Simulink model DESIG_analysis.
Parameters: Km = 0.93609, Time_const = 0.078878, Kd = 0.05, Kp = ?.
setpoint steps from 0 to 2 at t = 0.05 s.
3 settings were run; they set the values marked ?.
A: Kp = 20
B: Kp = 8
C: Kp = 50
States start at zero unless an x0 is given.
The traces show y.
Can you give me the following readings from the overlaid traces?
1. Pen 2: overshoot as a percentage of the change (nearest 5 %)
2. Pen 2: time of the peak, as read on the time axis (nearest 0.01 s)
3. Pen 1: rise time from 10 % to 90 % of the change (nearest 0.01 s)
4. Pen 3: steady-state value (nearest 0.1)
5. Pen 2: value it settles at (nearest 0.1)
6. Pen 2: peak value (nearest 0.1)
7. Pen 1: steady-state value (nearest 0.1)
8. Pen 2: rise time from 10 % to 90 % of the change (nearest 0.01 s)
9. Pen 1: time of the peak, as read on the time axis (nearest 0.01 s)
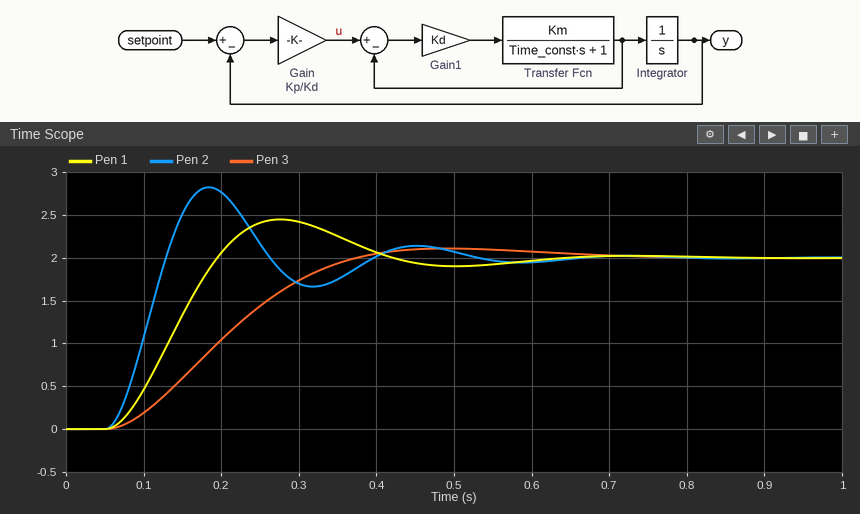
40 %
0.18 s
0.10 s
2.0
2.0
2.8
2.0
0.05 s
0.28 s
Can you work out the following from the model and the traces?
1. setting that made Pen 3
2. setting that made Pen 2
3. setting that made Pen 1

B
C
A
